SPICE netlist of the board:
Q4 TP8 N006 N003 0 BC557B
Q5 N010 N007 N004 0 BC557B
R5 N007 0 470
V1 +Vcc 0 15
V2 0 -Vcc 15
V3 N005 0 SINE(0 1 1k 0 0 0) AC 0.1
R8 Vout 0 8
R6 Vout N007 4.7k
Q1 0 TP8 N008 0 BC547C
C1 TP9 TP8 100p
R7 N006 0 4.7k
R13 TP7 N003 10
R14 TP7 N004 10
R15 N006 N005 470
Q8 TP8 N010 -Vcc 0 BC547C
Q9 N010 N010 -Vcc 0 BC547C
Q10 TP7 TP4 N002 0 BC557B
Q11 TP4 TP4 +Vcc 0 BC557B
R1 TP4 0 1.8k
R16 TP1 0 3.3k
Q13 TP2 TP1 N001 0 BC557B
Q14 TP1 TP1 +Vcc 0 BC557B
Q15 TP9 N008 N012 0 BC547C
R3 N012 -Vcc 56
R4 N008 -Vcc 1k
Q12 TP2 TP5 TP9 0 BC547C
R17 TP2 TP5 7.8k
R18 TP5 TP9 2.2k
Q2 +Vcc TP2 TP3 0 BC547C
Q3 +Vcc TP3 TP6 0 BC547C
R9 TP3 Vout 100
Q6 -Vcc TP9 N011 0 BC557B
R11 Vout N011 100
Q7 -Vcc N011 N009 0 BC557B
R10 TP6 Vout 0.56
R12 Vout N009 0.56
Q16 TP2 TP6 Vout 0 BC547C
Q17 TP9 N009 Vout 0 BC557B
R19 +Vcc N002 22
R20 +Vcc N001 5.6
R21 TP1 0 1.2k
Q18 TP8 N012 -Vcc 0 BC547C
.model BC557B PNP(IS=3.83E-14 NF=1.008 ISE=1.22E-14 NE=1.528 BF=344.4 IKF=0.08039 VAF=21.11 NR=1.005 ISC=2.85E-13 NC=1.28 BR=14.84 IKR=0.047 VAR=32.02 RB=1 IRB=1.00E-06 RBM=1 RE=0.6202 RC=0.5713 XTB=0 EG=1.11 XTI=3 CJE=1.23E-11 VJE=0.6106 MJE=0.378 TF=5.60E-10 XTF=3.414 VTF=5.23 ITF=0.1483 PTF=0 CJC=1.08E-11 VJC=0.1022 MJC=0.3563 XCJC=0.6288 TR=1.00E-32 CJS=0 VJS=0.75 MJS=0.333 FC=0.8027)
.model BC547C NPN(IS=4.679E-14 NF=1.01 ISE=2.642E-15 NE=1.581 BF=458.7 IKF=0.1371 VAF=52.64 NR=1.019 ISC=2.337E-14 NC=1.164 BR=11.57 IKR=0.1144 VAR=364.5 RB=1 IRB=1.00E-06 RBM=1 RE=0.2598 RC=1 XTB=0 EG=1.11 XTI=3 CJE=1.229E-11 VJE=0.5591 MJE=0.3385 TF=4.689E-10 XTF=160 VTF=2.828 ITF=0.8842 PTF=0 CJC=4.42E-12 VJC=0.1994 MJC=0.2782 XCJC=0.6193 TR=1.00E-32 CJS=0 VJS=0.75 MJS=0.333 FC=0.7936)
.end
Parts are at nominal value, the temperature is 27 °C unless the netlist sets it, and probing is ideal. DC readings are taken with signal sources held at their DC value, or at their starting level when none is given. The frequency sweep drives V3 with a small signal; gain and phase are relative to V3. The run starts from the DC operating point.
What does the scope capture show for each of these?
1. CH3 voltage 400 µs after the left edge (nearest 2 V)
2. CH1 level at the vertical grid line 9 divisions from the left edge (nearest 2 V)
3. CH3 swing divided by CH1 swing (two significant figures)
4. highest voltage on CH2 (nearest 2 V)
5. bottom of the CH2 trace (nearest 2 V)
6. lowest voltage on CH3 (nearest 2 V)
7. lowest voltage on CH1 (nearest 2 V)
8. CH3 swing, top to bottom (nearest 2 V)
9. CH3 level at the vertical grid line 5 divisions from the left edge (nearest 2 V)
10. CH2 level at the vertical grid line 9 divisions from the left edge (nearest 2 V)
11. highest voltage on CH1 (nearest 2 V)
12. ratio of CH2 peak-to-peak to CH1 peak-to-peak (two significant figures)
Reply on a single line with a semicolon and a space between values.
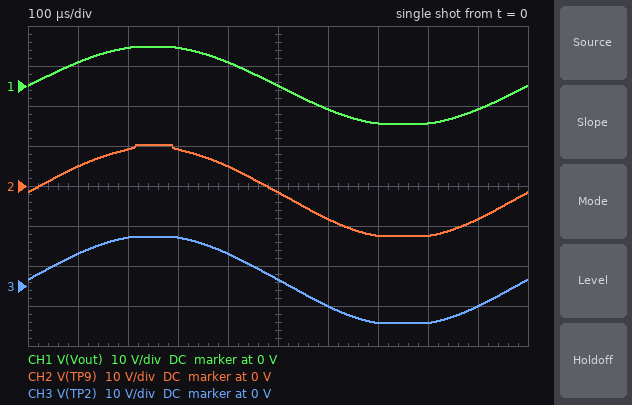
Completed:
8 V; -6 V; 1.1; 10 V; -12 V; -10 V; -10 V; 22 V; 2 V; -8 V; 10 V; 1.2
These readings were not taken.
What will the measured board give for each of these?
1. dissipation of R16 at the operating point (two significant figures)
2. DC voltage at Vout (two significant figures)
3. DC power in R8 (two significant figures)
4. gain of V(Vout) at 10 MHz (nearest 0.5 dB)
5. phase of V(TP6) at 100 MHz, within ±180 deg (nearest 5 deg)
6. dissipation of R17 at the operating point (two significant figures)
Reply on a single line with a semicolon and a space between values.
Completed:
62 mW; 17 mV; 37 µW; 11.5 dB; 5 deg; 810 µW
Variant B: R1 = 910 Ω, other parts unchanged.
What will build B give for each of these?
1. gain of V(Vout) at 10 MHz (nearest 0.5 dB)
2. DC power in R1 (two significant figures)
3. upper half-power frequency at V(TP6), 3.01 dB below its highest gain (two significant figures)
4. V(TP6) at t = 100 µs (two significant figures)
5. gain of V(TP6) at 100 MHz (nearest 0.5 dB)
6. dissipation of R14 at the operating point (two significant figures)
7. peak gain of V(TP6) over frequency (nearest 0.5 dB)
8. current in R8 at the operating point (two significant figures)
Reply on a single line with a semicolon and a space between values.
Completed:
13.5 dB; 220 mW; 7.2 MHz; 6.3 V; -25.0 dB; 23 µW; 22.0 dB; 2.2 mA
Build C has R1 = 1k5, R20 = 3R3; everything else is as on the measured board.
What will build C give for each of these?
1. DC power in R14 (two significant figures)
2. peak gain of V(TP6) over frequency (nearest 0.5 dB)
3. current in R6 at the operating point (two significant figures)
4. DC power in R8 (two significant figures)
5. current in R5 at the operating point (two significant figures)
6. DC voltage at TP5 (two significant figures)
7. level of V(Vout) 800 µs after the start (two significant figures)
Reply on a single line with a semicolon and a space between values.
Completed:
14 µW; 20.5 dB; 8.2 µA; 240 µW; 10 µA; -940 mV; -8.6 V
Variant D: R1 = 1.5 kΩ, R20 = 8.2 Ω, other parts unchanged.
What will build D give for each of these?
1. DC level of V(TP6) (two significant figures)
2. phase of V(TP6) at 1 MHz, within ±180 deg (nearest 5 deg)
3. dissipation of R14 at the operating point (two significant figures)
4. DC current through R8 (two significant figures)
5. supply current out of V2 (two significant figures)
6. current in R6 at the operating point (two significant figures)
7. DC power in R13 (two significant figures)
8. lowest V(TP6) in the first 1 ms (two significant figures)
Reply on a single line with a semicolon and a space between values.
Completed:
89 mV; -15 deg; 15 µW; 1.9 mA; 150 mA; 2.8 µA; 16 µW; -9.7 V
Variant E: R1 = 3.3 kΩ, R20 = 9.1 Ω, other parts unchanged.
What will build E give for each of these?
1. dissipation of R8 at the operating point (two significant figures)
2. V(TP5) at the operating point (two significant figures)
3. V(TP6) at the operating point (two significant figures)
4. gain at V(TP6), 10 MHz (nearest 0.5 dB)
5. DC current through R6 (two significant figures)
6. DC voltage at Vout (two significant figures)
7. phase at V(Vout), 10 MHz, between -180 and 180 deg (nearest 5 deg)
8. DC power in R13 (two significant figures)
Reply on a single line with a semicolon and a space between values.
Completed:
27 µW; -900 mV; 85 mV; 10.0 dB; 2.7 µA; 15 mV; -170 deg; 8.0 µW
